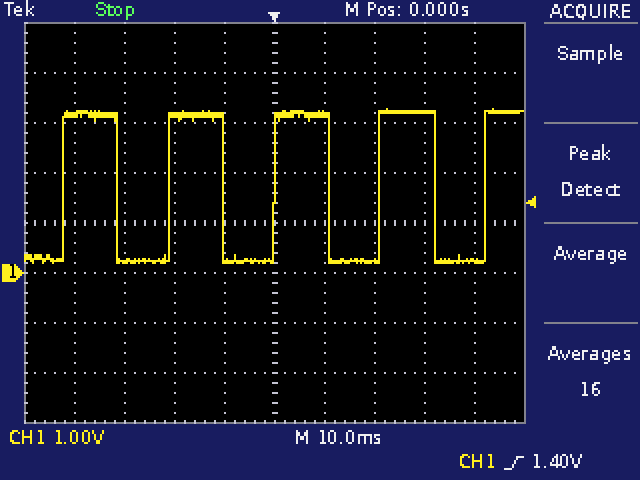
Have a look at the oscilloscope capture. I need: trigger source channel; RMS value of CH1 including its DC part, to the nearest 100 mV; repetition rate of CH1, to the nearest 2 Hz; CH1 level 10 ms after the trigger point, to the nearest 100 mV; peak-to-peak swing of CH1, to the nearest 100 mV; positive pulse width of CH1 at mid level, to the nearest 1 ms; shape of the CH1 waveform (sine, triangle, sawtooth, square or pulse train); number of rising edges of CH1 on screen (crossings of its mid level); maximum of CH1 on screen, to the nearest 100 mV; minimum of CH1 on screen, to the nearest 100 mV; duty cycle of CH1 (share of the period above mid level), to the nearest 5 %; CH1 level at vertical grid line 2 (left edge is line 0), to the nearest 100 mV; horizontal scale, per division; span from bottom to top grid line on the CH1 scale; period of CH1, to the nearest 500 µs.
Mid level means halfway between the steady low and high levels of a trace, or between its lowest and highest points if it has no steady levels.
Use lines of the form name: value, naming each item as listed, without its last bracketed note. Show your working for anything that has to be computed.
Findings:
trigger source channel: CH1
RMS value of CH1 including its DC part, to the nearest 100 mV: √(0.5 × (3.3 V)² + 0.5 × (200 mV)²) ≈ 2.3 V
repetition rate of CH1, to the nearest 2 Hz: 1 / 21.0 ms ≈ 48 Hz
CH1 level 10 ms after the trigger point, to the nearest 100 mV: 3.2 V
peak-to-peak swing of CH1, to the nearest 100 mV: 3.3 V − (200 mV) = 3.1 V
positive pulse width of CH1 at mid level, to the nearest 1 ms: 11 ms
shape of the CH1 waveform: square
number of rising edges of CH1 on screen: 5
maximum of CH1 on screen, to the nearest 100 mV: 3.3 V
minimum of CH1 on screen, to the nearest 100 mV: 200 mV
duty cycle of CH1 (share of the period above mid level), to the nearest 5 %: 11 ms / 21.0 ms ≈ 52.4 %, so 50 % to the nearest 5 %
CH1 level at vertical grid line 2 (left edge is line 0), to the nearest 100 mV: 200 mV
horizontal scale, per division: 10 ms
span from bottom to top grid line on the CH1 scale: 8 V
period of CH1, to the nearest 500 µs: 21.0 ms
